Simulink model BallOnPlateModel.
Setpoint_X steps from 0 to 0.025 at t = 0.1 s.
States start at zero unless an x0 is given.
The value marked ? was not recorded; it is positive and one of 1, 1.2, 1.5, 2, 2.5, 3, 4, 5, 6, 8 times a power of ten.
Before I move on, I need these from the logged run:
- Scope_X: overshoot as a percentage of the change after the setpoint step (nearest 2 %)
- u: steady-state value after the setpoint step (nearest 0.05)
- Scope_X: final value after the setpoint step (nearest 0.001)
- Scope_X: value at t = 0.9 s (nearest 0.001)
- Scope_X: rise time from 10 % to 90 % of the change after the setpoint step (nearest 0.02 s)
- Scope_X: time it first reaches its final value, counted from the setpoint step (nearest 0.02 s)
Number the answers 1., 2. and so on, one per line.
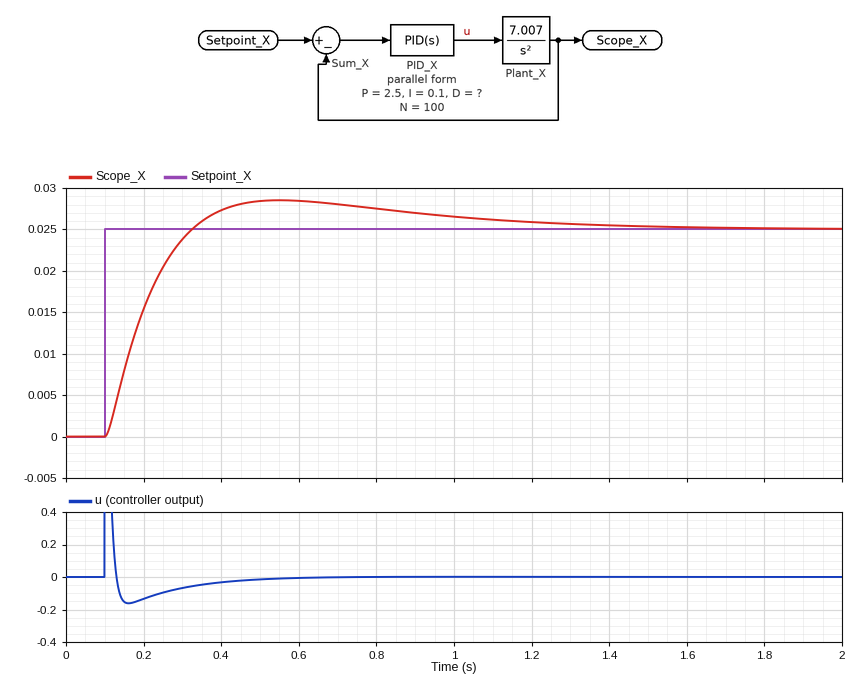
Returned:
1. 14 %
2. 0.00
3. 0.025
4. 0.027
5. 0.16 s
6. 0.22 s
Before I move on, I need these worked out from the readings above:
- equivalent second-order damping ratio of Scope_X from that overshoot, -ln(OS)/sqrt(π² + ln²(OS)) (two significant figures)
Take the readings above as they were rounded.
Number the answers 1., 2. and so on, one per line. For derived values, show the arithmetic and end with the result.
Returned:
1. ln(0.14) = -1.966; 1.966 / sqrt(9.870 + 3.866) = 0.53
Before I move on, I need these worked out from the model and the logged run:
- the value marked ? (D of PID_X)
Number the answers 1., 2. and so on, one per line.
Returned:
1. 1.2
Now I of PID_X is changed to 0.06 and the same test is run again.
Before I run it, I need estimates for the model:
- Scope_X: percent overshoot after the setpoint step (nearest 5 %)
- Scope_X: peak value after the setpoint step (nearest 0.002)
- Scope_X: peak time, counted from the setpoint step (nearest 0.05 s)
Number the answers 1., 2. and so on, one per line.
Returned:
1. 15 %
2. 0.028
3. 0.45 s
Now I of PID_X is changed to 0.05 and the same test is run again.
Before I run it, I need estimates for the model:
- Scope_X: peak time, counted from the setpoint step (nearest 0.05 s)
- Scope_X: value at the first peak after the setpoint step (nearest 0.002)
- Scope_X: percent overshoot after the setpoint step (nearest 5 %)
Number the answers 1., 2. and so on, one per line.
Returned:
1. 0.45 s
2. 0.028
3. 15 %
